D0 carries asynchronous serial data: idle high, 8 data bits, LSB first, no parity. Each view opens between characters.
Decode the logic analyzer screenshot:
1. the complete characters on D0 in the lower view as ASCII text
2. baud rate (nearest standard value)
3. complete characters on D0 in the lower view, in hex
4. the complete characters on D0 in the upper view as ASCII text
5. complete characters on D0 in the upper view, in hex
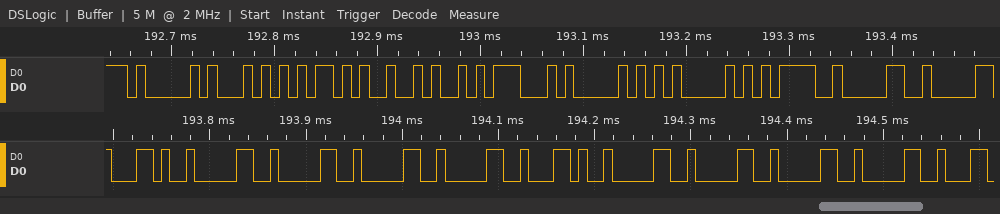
",0000,0000"
115200 baud
2C, 30, 30, 30, 30, 2C, 30, 30, 30, 30
"AT+JGPA=0"
41, 54, 2B, 4A, 47, 50, 41, 3D, 30
